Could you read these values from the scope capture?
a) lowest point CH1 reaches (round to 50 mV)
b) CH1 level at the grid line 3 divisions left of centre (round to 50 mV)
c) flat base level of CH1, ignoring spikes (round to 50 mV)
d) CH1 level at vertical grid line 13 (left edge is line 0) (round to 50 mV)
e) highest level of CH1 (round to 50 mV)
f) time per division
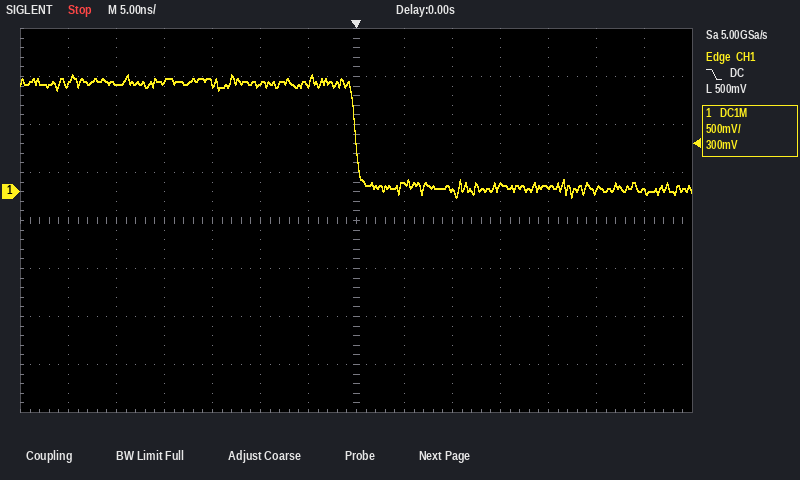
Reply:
-50 mV
1.15 V
50 mV
0 mV
1.20 V
5 ns
